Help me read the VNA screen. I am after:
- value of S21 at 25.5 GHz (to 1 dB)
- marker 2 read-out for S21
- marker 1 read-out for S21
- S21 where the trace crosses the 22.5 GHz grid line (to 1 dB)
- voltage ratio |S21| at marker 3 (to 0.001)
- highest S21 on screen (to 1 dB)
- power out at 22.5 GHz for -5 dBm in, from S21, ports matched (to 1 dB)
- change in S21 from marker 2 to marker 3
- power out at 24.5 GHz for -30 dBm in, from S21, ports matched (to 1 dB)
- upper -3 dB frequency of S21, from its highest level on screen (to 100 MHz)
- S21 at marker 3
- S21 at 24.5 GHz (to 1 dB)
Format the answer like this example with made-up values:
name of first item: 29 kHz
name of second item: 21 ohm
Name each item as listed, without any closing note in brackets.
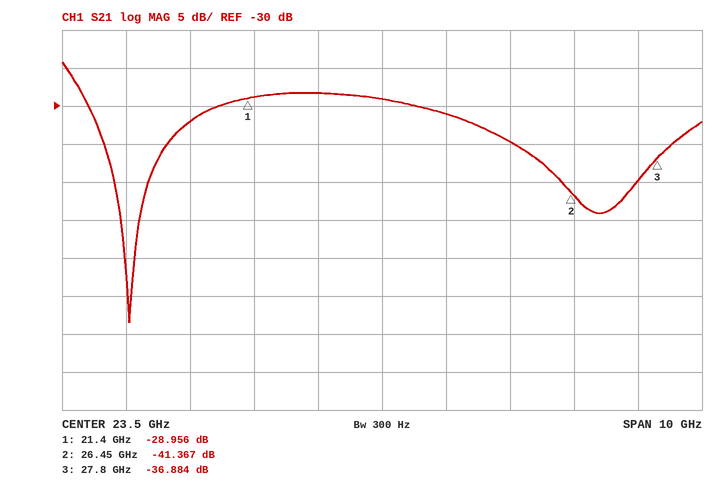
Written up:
value of S21 at 25.5 GHz: -35 dB
marker 2 read-out for S21: -41.367 dB
marker 1 read-out for S21: -28.956 dB
S21 where the trace crosses the 22.5 GHz grid line: -28 dB
voltage ratio |S21| at marker 3: 0.014
highest S21 on screen: -24 dB
power out at 22.5 GHz for -5 dBm in, from S21, ports matched: -33 dBm
change in S21 from marker 2 to marker 3: 4.483 dB
power out at 24.5 GHz for -30 dBm in, from S21, ports matched: -61 dBm
upper -3 dB frequency of S21, from its highest level on screen: 18.7 GHz
S21 at marker 3: -36.884 dB
S21 at 24.5 GHz: -31 dB
